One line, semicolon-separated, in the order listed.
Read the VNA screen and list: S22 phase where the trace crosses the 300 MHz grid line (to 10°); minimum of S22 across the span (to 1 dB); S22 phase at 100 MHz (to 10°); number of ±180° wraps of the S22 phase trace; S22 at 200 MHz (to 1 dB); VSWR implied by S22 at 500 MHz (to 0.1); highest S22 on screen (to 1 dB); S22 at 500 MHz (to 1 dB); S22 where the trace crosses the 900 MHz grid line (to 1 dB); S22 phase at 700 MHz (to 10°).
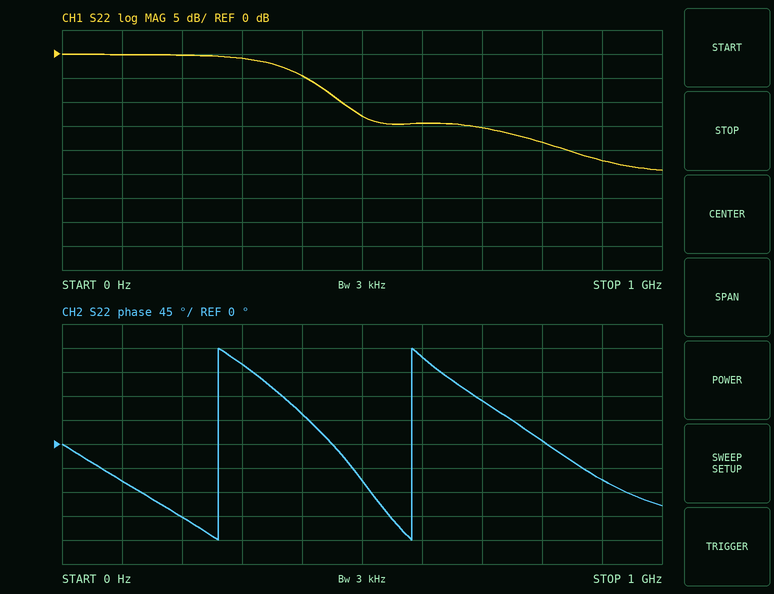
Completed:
150°; -24 dB; -70°; 2; 0 dB; 1.6; 0 dB; -13 dB; -22 dB; 80°
